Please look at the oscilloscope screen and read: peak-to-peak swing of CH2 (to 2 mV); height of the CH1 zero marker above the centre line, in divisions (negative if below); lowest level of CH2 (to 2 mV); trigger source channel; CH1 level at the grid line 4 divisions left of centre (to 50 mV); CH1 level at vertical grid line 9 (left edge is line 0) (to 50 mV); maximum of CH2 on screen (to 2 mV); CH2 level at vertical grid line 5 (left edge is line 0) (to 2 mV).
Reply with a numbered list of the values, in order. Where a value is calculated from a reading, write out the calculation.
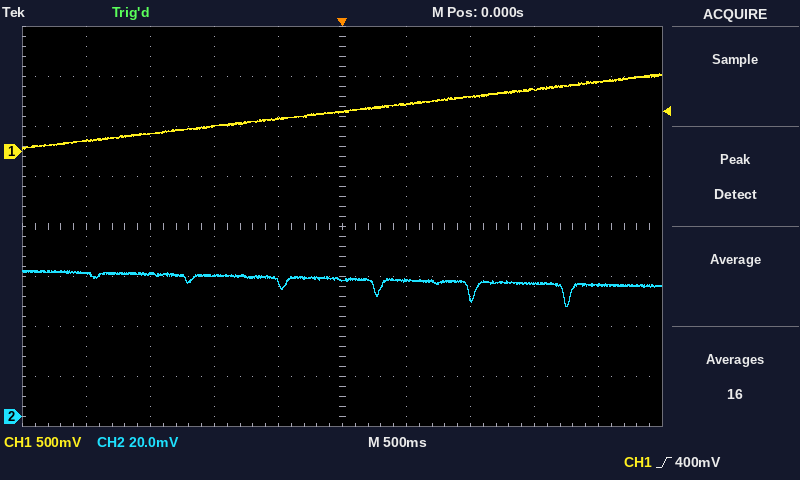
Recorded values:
1. 58 mV − (44 mV) = 14 mV
2. +1.5 div
3. 44 mV
4. CH1
5. 100 mV
6. 700 mV
7. 58 mV
8. 54 mV
